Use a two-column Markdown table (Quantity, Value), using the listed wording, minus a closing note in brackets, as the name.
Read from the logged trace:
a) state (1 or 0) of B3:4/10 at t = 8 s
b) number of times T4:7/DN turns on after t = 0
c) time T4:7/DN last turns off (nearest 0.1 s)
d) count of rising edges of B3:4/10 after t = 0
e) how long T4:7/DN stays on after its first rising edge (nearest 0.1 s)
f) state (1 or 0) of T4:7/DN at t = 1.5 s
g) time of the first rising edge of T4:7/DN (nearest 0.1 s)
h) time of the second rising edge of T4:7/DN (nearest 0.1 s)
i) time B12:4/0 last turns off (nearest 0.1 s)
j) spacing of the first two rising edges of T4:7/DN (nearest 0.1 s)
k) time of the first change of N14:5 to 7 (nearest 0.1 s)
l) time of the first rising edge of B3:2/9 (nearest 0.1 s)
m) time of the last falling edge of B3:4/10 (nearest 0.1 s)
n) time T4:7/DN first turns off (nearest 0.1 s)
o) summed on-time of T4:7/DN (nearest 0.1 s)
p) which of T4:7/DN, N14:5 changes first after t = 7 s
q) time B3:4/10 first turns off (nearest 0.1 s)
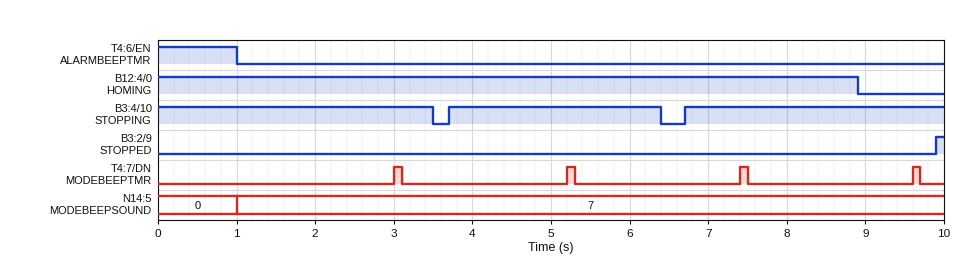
| Quantity | Value |
|---|---|
| state (1 or 0) of B3:4/10 at t = 8 s | 1 |
| number of times T4:7/DN turns on after t = 0 | 4 |
| time T4:7/DN last turns off | 9.7 s |
| count of rising edges of B3:4/10 after t = 0 | 2 |
| how long T4:7/DN stays on after its first rising edge | 0.1 s |
| state (1 or 0) of T4:7/DN at t = 1.5 s | 0 |
| time of the first rising edge of T4:7/DN | 3.0 s |
| time of the second rising edge of T4:7/DN | 5.2 s |
| time B12:4/0 last turns off | 8.9 s |
| spacing of the first two rising edges of T4:7/DN | 2.2 s |
| time of the first change of N14:5 to 7 | 1.0 s |
| time of the first rising edge of B3:2/9 | 9.9 s |
| time of the last falling edge of B3:4/10 | 6.4 s |
| time T4:7/DN first turns off | 3.1 s |
| summed on-time of T4:7/DN | 0.4 s |
| which of T4:7/DN, N14:5 changes first after t = 7 s | T4:7/DN |
| time B3:4/10 first turns off | 3.5 s |
